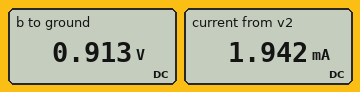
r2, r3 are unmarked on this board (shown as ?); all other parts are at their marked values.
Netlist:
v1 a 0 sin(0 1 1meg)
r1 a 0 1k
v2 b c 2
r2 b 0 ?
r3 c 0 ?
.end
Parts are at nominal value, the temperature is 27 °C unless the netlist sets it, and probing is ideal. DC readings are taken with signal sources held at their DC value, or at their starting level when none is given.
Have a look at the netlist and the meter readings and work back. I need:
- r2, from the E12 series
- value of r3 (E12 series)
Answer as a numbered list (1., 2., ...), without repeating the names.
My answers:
1. 470 Ω
2. 560 Ω
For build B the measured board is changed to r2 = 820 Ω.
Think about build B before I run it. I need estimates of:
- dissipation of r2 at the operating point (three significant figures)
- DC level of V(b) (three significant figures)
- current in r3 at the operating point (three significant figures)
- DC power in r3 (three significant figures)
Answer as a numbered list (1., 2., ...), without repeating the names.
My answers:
1. 1.72 mW
2. 1.19 V
3. 1.45 mA
4. 1.18 mW
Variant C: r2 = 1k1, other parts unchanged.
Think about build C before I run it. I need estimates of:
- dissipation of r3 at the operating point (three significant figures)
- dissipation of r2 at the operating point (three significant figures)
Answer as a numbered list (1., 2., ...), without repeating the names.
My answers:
1. 813 µW
2. 1.60 mW
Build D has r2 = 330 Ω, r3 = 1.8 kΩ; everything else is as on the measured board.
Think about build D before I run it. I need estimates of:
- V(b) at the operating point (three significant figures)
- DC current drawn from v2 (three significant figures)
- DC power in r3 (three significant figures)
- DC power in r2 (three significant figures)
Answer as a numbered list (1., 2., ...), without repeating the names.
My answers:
1. 310 mV
2. 939 µA
3. 1.59 mW
4. 291 µW
